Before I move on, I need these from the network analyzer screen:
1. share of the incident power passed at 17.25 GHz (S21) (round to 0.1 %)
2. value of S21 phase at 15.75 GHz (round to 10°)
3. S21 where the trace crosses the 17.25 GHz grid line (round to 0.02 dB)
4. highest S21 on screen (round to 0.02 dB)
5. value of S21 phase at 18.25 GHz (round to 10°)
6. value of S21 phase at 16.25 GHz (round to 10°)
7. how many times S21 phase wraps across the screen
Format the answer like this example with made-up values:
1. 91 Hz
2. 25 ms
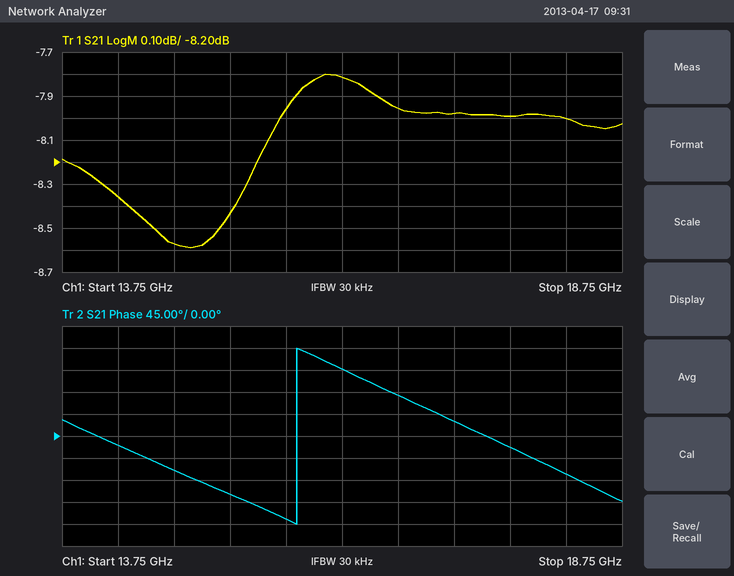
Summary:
1. 15.9 %
2. -170°
3. -7.98 dB
4. -7.80 dB
5. -80°
6. 140°
7. 1
